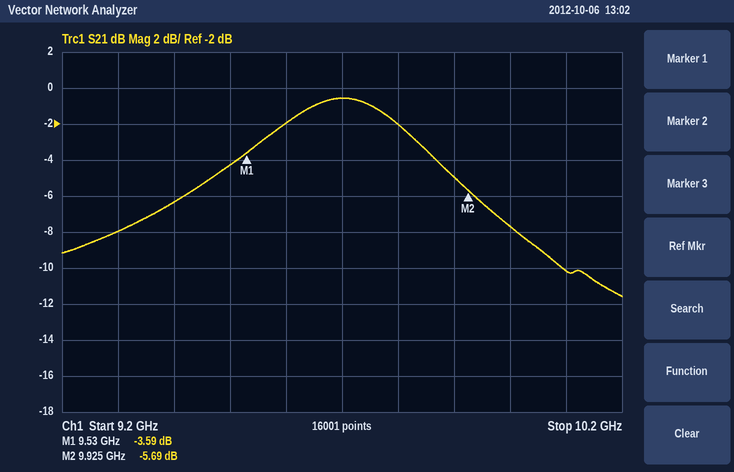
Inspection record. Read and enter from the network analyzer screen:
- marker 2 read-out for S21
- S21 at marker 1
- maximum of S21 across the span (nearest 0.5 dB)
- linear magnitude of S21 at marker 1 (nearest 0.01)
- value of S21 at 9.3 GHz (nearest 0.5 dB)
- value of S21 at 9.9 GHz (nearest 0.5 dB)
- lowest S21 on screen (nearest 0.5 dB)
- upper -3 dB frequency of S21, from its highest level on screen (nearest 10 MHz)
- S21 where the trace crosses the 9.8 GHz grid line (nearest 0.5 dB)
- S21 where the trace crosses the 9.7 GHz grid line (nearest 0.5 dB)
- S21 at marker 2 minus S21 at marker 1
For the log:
-5.69 dB
-3.59 dB
-0.5 dB
0.66
-8.0 dB
-5.0 dB
-11.5 dB
9.85 GHz
-2.0 dB
-0.5 dB
-2.10 dB
